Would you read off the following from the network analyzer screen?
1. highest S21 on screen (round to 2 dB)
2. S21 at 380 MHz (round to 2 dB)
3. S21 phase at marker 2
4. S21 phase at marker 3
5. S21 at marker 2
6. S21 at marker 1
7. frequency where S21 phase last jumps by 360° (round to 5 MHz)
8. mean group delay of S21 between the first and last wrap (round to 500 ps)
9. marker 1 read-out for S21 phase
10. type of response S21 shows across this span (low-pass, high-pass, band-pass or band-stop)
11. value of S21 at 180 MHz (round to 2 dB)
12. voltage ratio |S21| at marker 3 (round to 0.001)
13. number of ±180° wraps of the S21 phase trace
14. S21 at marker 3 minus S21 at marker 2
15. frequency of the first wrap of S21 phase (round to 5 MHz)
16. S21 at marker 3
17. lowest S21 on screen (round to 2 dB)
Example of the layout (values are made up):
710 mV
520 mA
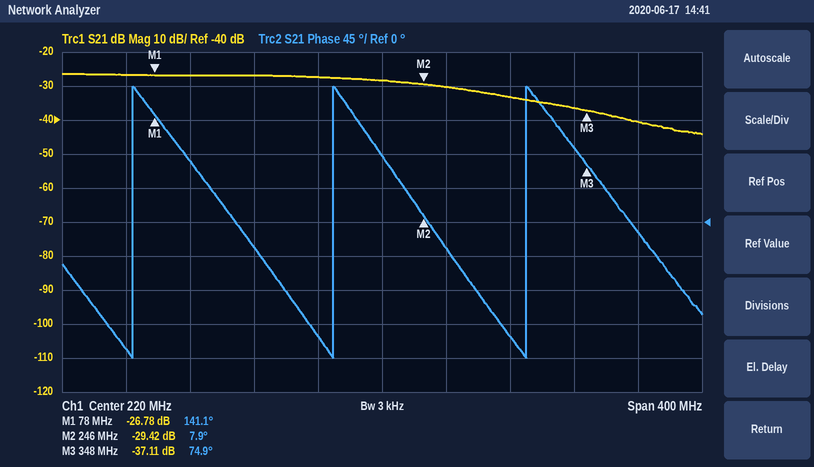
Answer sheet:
-26 dB
-40 dB
7.9°
74.9°
-29.42 dB
-26.78 dB
310 MHz
8.0 ns
141.1°
low-pass
-28 dB
0.014
3
-7.69 dB
65 MHz
-37.11 dB
-44 dB
